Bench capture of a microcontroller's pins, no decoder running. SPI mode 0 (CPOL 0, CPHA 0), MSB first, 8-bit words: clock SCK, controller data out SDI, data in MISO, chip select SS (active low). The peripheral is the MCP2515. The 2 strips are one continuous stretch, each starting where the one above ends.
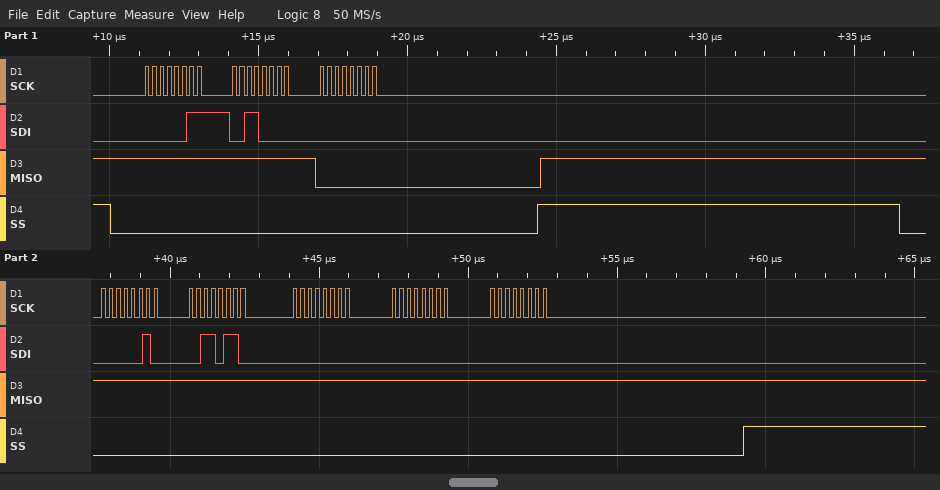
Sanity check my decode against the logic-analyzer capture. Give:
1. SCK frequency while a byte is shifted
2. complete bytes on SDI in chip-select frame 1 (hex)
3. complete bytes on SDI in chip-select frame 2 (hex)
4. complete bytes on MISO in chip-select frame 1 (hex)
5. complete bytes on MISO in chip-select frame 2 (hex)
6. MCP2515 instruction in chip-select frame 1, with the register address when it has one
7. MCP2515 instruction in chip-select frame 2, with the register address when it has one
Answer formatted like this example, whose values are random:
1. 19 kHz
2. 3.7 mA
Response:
1. 4 MHz
2. 03 30 00
3. 02 36 00 00 00
4. FF FF 00
5. FF FF FF FF FF
6. READ 0x30
7. WRITE 0x36
